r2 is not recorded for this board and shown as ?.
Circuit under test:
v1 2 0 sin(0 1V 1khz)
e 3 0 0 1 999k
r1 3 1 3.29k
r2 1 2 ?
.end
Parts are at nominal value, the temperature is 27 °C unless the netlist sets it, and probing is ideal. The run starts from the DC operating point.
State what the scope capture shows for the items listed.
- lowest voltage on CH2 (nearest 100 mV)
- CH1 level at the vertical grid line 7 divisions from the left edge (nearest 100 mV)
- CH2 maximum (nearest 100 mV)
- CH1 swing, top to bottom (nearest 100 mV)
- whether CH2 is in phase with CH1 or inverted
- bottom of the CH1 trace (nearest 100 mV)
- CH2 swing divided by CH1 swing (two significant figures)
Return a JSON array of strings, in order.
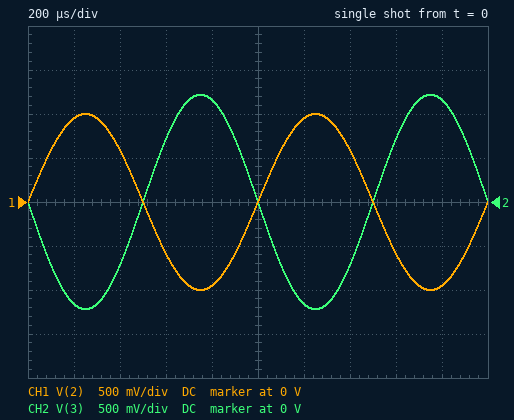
["-1.2 V", "600 mV", "1.2 V", "2.0 V", "inverted", "-1.0 V", "1.2"]
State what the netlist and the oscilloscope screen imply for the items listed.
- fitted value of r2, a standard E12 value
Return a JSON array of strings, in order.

["2.7 kΩ"]
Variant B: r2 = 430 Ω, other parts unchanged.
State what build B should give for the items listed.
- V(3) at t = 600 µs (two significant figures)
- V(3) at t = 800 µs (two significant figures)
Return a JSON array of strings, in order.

["4.5 V", "7.3 V"]
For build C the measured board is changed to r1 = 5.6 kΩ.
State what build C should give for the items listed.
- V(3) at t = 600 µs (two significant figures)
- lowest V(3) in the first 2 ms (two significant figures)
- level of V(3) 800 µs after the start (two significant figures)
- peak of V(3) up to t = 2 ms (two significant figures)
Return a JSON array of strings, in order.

["1.2 V", "-2.1 V", "2.0 V", "2.1 V"]
